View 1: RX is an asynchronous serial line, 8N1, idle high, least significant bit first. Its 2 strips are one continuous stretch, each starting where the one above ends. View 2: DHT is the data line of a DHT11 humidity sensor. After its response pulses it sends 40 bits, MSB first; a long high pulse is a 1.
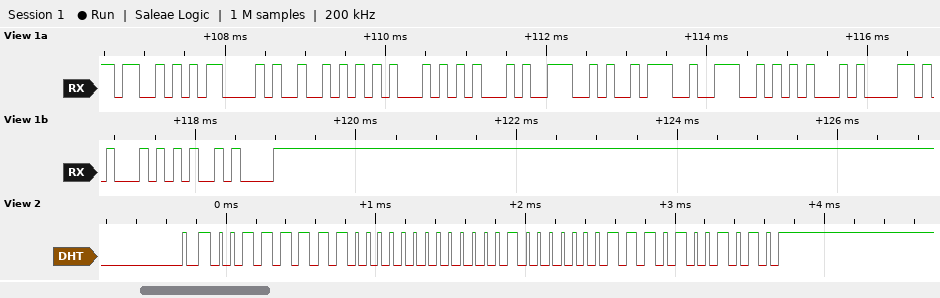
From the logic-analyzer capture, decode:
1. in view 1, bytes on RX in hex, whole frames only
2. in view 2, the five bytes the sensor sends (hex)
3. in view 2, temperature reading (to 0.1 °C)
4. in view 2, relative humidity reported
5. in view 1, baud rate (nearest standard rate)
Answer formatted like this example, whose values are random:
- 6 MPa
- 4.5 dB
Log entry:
- 53 43 52 45 45 4E 3A 4E 45 58 54 0A
- 3F 00 04 07 4A
- 4.7 °C
- 63 %
- 9600 baud
